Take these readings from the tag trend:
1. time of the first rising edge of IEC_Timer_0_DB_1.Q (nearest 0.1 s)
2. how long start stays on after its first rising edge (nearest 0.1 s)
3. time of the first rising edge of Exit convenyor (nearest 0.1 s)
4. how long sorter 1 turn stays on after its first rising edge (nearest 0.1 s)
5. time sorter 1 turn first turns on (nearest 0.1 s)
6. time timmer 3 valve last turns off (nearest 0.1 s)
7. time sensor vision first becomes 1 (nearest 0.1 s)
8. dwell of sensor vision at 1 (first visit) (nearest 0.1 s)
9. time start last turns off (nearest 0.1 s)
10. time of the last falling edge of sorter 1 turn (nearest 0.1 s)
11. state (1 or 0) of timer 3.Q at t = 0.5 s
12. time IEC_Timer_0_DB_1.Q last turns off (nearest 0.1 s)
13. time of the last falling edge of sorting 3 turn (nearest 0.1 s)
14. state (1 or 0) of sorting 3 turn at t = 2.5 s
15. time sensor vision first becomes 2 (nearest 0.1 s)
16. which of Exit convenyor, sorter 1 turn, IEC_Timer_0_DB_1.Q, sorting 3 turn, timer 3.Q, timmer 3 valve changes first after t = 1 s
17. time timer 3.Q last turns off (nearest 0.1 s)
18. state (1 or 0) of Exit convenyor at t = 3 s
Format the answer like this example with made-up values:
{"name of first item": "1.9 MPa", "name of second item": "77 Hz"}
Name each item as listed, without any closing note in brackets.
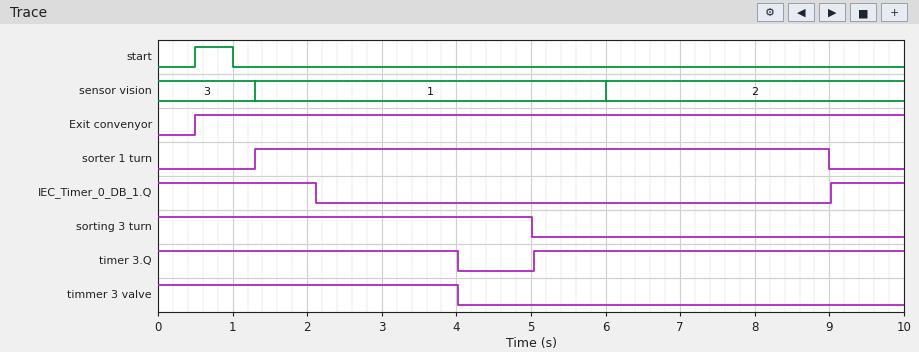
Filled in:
{"time of the first rising edge of IEC_Timer_0_DB_1.Q": "9.0 s", "how long start stays on after its first rising edge": "0.5 s", "time of the first rising edge of Exit convenyor": "0.5 s", "how long sorter 1 turn stays on after its first rising edge": "7.7 s", "time sorter 1 turn first turns on": "1.3 s", "time timmer 3 valve last turns off": "4.0 s", "time sensor vision first becomes 1": "1.3 s", "dwell of sensor vision at 1 (first visit)": "4.7 s", "time start last turns off": "1.0 s", "time of the last falling edge of sorter 1 turn": "9.0 s", "state (1 or 0) of timer 3.Q at t = 0.5 s": "1", "time IEC_Timer_0_DB_1.Q last turns off": "2.1 s", "time of the last falling edge of sorting 3 turn": "5.0 s", "state (1 or 0) of sorting 3 turn at t = 2.5 s": "1", "time sensor vision first becomes 2": "6.0 s", "which of Exit convenyor, sorter 1 turn, IEC_Timer_0_DB_1.Q, sorting 3 turn, timer 3.Q, timmer 3 valve changes first after t = 1 s": "sorter 1 turn", "time timer 3.Q last turns off": "4.0 s", "state (1 or 0) of Exit convenyor at t = 3 s": "1"}
